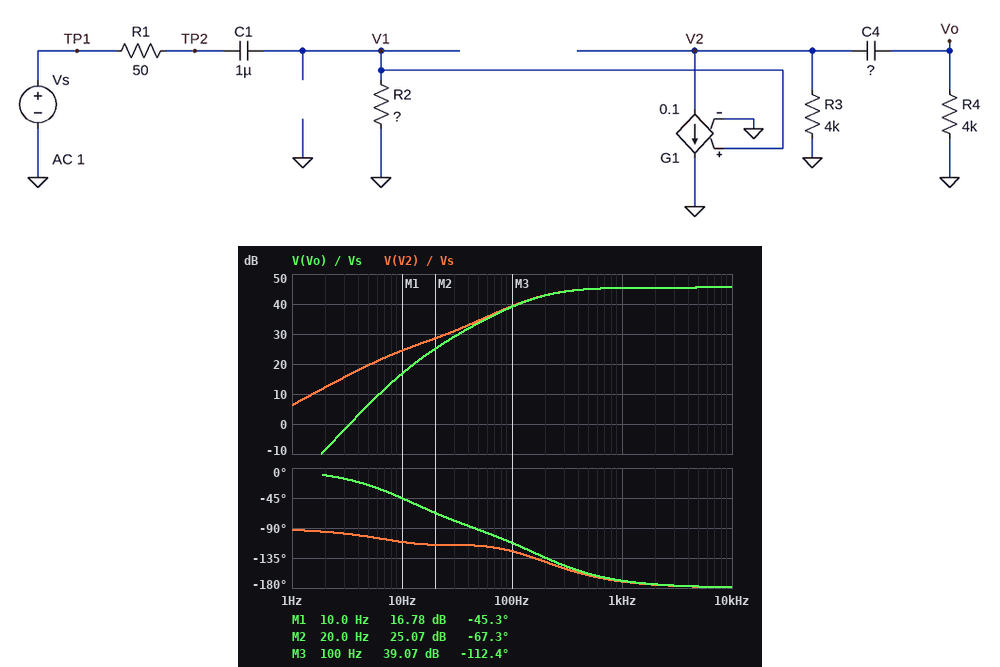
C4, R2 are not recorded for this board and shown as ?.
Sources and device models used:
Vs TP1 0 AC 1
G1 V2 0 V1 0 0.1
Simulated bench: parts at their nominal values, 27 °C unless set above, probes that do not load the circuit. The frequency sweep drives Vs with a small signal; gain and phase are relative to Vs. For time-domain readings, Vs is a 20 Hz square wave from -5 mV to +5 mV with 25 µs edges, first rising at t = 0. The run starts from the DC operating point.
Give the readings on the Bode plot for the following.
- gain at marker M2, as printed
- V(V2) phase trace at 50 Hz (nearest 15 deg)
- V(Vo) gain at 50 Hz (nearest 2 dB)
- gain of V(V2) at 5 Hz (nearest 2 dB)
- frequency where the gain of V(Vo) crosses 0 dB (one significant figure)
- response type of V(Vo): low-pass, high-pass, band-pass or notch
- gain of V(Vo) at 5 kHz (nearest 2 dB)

25.07 dB
-120 deg
34 dB
20 dB
3 Hz
high-pass
46 dB
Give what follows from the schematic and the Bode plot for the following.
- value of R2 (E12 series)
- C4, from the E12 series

820 Ω
1.8 µF
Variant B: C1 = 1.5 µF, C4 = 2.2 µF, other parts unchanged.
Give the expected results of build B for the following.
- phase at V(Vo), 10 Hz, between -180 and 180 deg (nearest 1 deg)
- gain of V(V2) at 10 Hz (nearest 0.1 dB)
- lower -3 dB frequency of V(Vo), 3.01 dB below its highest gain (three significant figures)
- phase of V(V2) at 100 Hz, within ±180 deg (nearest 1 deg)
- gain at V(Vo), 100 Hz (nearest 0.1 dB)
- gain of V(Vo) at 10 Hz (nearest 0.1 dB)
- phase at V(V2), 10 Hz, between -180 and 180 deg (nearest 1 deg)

-53 deg
27.5 dB
123 Hz
-134 deg
41.5 dB
21.2 dB
-114 deg
